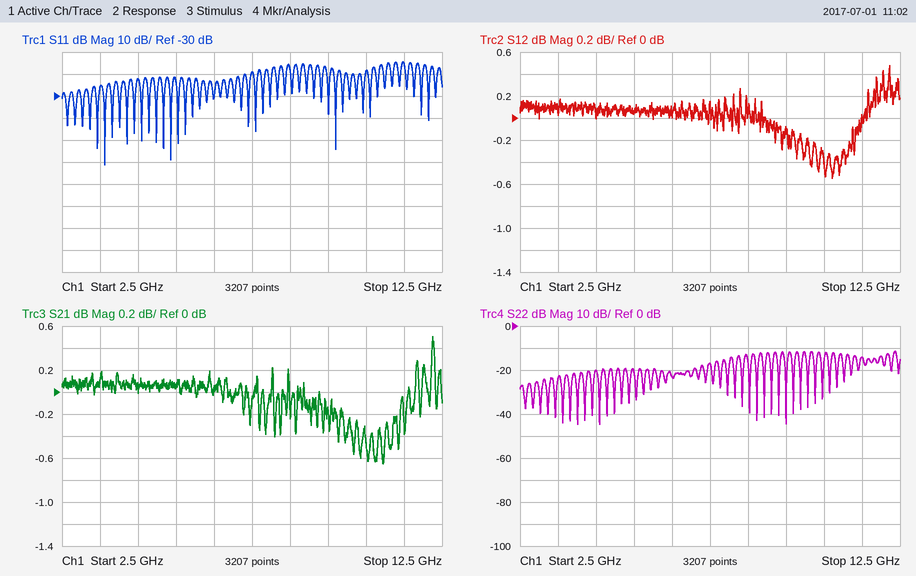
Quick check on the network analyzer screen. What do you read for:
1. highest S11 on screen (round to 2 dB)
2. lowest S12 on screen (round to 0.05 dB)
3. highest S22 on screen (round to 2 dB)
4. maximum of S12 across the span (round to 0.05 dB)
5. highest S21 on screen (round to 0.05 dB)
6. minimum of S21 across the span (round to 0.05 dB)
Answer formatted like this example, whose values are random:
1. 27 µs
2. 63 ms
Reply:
1. -14 dB
2. -0.55 dB
3. -12 dB
4. 0.50 dB
5. 0.50 dB
6. -0.65 dB
